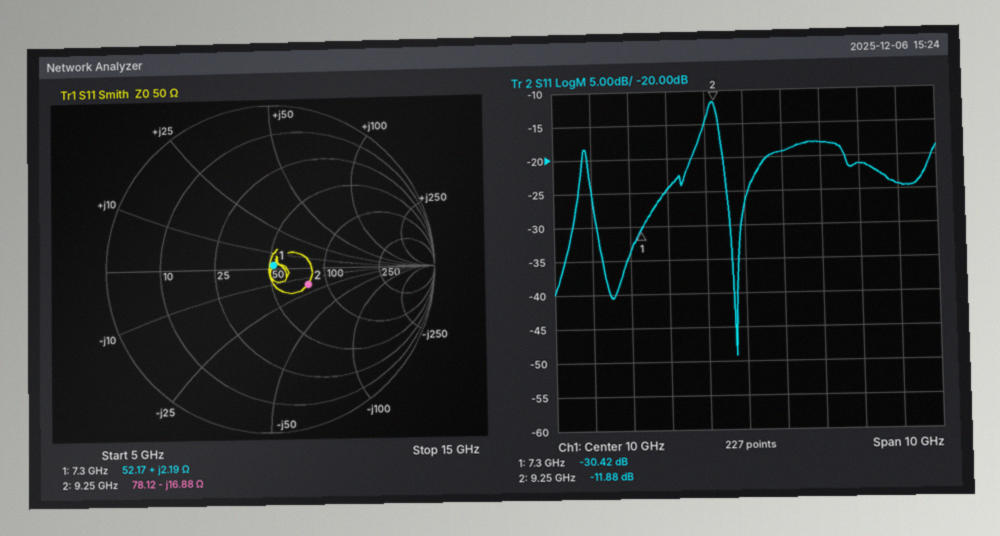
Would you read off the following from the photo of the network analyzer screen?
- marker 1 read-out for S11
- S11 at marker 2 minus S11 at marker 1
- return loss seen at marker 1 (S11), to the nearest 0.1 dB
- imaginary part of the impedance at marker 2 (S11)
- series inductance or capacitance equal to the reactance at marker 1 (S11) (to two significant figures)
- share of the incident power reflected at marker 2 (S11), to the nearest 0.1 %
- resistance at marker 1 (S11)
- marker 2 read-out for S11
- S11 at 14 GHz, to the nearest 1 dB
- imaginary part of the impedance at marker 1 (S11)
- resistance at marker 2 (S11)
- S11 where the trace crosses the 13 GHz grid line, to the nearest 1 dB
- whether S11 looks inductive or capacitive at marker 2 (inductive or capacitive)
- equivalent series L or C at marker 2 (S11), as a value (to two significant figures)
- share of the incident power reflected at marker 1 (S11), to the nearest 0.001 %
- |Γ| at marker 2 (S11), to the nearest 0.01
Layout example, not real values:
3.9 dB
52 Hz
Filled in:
-30.42 dB
18.54 dB
30.4 dB
-16.88 Ω
48 pH
6.5 %
52.17 Ω
-11.88 dB
-24 dB
+2.19 Ω
78.12 Ω
-21 dB
capacitive
1.0 pF
0.091 %
0.25
